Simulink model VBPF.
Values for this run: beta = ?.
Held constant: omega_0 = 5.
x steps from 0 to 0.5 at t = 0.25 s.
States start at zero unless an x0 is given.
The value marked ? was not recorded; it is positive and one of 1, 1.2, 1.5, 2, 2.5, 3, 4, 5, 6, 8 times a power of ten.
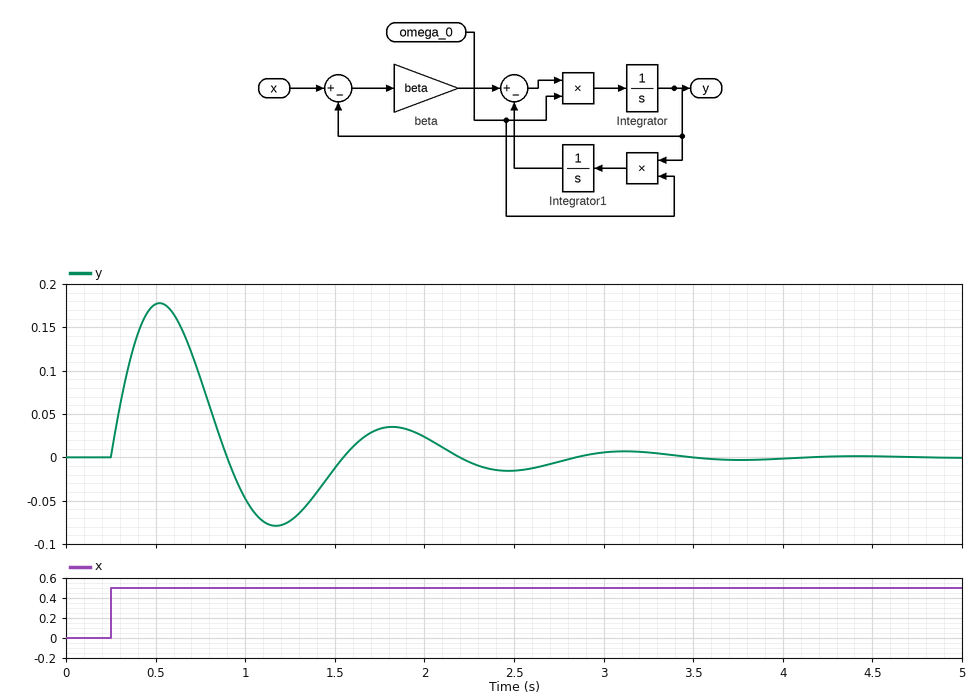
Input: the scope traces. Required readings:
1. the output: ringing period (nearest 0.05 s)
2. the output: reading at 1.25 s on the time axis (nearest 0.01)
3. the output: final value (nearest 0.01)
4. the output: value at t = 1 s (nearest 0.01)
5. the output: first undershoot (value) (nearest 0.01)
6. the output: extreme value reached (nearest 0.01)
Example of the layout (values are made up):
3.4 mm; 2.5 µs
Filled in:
1.30 s; -0.07; 0.00; -0.05; -0.08; 0.18
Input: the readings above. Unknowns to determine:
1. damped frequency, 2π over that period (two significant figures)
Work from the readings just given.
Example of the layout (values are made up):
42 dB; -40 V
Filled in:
4.8 rad/s
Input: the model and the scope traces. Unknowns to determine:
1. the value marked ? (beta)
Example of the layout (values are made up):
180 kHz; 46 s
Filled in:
0.5
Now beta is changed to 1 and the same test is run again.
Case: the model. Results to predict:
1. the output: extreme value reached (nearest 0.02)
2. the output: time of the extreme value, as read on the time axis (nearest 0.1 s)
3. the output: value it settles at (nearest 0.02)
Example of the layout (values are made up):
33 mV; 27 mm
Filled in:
0.28; 0.5 s; 0.00
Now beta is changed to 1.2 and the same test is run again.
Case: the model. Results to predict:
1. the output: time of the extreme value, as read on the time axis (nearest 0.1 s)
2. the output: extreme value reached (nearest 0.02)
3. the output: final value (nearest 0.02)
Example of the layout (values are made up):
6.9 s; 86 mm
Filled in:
0.5 s; 0.30; 0.00
